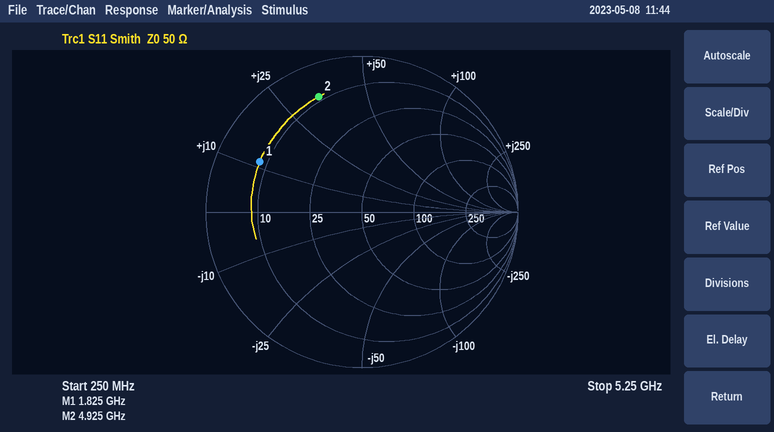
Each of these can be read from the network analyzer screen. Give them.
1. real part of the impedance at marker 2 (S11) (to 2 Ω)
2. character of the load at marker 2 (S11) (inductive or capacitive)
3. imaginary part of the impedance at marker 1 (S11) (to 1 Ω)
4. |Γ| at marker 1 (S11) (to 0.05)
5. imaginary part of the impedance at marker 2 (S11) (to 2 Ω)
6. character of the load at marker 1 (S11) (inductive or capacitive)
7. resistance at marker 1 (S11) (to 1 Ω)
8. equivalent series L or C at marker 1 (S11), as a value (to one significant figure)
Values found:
8 Ω
inductive
+11 Ω
0.75
+34 Ω
inductive
8 Ω
1.0 nH
